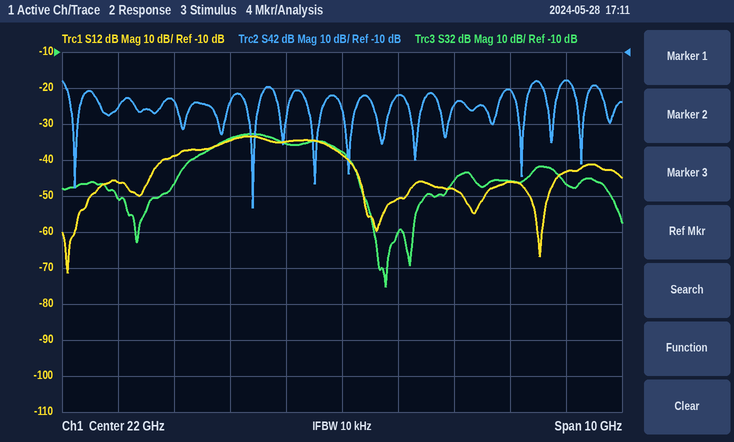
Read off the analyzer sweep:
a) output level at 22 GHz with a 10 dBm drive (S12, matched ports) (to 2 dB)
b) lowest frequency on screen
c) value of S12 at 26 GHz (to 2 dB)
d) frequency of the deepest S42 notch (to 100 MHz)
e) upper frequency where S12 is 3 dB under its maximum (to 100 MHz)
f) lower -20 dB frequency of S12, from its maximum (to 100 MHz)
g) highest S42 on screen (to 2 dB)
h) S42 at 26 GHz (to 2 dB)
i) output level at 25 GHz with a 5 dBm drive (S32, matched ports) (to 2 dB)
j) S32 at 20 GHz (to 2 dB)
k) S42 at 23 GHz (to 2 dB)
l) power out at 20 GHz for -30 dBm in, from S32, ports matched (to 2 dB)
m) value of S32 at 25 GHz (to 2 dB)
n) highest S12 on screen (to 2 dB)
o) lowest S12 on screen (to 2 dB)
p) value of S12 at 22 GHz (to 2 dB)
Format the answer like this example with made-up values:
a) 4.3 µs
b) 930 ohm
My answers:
a) -28 dBm
b) 17 GHz
c) -44 dB
d) 20.4 GHz
e) 21.8 GHz
f) 17.4 GHz
g) -18 dB
h) -18 dB
i) -40 dBm
j) -34 dB
k) -22 dB
l) -64 dBm
m) -46 dB
n) -34 dB
o) -72 dB
p) -38 dB
